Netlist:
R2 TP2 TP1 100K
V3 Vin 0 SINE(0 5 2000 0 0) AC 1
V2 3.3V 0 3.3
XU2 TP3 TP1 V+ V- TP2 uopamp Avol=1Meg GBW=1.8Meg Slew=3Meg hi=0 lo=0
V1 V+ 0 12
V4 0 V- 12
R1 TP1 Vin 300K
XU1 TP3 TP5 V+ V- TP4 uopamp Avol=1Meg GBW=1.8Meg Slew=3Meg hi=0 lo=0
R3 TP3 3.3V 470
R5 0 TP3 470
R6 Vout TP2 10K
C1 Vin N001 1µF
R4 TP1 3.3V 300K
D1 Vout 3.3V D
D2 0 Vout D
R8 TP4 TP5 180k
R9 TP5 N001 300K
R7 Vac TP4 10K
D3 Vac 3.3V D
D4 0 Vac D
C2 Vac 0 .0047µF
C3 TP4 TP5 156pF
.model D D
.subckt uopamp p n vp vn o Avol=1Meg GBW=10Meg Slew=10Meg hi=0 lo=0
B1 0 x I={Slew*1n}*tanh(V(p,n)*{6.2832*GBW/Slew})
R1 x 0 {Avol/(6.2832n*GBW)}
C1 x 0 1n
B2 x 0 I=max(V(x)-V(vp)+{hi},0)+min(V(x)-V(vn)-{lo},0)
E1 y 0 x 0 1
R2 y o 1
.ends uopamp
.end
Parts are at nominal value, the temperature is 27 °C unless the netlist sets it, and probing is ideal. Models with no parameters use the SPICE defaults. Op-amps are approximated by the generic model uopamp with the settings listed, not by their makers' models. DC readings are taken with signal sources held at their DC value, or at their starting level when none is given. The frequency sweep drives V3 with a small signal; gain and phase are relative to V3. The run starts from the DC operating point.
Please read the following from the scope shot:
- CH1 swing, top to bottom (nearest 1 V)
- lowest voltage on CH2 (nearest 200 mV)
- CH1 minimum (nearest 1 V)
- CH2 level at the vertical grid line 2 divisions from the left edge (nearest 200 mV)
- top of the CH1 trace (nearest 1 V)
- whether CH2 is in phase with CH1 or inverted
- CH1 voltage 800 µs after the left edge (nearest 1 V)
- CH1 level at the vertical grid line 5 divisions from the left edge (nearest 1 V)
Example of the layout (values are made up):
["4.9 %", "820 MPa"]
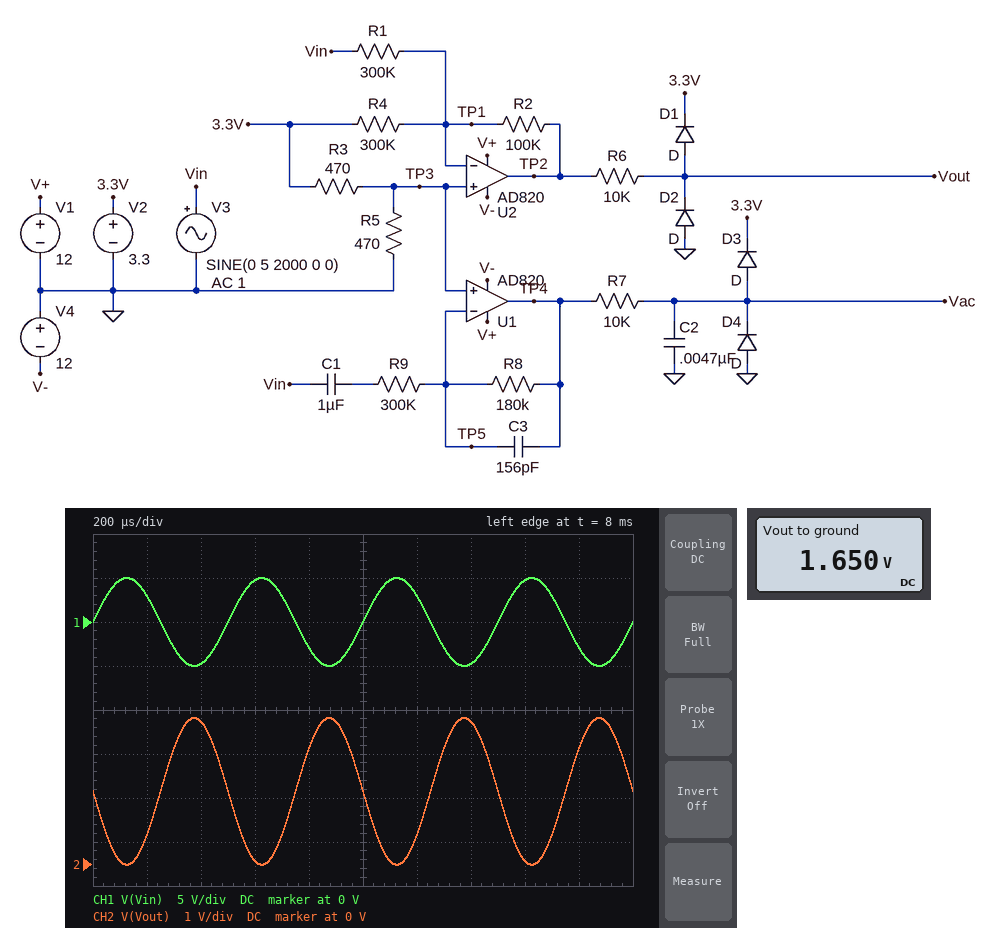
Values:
["10 V", "0 V", "-5 V", "3.2 V", "5 V", "inverted", "-3 V", "0 V"]
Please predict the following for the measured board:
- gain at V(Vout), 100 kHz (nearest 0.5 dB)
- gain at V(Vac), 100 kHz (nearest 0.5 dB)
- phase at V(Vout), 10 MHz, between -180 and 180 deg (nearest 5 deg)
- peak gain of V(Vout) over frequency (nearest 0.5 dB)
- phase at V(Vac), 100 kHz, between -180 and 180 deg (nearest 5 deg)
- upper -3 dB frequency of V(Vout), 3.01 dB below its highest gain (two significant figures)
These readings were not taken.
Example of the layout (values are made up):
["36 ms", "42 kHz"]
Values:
["-9.5 dB", "-59.0 dB", "95 deg", "-9.5 dB", "0 deg", "1.1 MHz"]
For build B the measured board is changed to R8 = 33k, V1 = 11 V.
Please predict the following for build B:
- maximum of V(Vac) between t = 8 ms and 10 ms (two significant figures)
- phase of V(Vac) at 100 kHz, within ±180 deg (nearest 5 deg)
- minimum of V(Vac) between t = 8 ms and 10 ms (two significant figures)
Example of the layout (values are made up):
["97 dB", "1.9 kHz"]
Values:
["2.1 V", "15 deg", "1.2 V"]
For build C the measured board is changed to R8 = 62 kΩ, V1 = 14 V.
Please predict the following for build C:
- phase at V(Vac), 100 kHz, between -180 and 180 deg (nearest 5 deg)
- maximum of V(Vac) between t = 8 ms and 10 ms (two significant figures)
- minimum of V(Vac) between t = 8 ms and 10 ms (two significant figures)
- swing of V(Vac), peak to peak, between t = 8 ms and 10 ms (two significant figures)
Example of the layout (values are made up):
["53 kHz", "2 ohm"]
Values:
["10 deg", "2.5 V", "770 mV", "1.8 V"]
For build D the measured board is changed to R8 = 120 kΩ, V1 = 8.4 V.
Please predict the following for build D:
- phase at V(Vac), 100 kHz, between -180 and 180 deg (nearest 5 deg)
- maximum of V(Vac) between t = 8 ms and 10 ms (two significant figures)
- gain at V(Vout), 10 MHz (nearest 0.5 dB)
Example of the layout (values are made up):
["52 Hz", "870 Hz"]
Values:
["5 deg", "3.3 V", "-29.0 dB"]
